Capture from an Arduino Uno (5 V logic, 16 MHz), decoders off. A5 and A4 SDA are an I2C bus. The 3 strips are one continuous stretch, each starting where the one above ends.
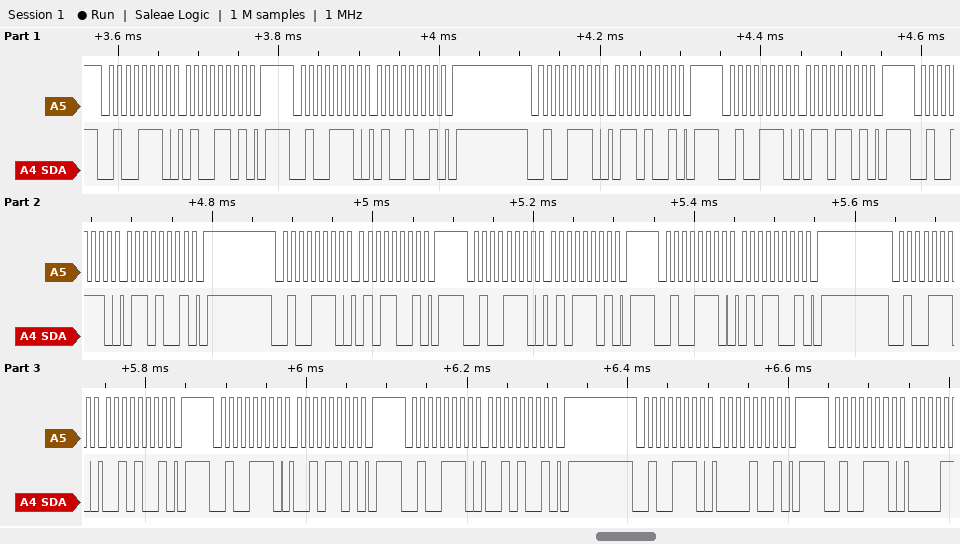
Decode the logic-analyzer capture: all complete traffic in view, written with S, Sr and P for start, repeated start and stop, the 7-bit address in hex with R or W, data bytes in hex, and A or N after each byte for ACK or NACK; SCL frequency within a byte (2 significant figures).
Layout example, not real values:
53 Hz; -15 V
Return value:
S 27W A 4D A P S 27W A 49 A P S 27W A 69 A P S 27W A 6D A P S 27W A 69 A P S 27W A 59 A P S 27W A 5D A P S 27W A 59 A P S 27W A 29 A P S 27W A 2D A P S 27W A 29 A P S 27W A 09 A P S 27W A; 100 kHz
